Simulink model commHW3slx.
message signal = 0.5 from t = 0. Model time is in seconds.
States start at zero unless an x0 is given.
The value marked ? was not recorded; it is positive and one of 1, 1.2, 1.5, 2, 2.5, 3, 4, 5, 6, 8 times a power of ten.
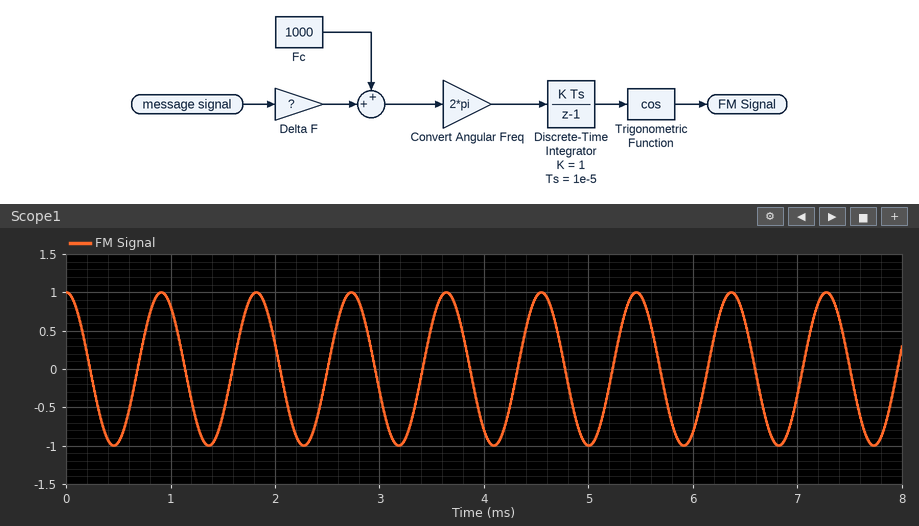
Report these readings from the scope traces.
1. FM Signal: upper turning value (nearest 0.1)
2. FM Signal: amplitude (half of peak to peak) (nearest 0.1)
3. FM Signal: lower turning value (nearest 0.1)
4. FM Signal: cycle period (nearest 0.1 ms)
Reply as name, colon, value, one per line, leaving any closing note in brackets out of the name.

FM Signal: upper turning value: 1.0
FM Signal: amplitude (half of peak to peak): 1.0
FM Signal: lower turning value: -1.0
FM Signal: cycle period: 0.9 ms
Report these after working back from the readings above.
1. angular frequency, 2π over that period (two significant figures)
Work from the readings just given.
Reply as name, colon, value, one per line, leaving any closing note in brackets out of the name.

angular frequency, 2π over that period: 7.0 rad/ms
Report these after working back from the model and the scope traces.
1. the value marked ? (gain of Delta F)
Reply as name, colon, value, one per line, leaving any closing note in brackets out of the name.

the value marked ?: 200
